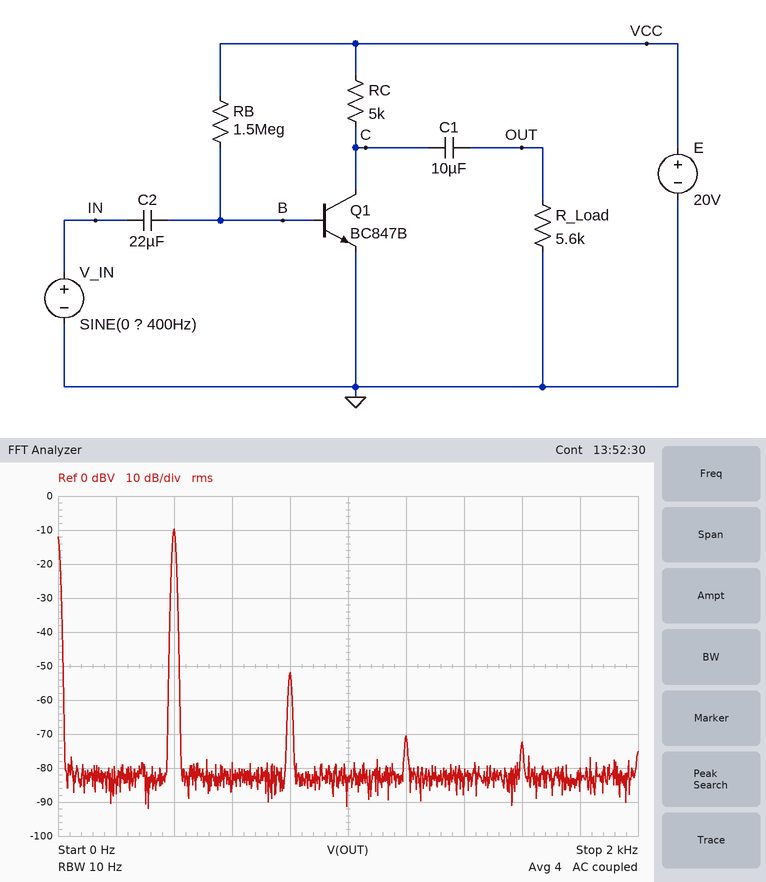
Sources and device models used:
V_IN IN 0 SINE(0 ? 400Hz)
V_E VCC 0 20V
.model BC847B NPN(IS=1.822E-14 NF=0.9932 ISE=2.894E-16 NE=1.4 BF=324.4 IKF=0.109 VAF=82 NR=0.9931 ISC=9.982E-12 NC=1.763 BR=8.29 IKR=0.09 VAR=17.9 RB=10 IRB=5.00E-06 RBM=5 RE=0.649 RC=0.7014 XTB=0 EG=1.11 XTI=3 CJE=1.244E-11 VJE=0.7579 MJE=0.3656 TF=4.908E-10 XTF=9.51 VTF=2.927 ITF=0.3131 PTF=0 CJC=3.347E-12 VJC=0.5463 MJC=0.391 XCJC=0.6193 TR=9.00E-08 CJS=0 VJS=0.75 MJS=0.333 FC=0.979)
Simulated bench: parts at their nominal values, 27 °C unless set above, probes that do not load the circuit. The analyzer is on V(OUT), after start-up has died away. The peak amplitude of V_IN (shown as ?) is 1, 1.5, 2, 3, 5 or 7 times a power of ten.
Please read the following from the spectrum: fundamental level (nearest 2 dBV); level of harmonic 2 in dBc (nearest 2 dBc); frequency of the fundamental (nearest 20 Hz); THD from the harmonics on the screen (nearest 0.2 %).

-10 dBV
-42 dBc
400 Hz
0.8 %
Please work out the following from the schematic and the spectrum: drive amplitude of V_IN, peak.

1.5 mV
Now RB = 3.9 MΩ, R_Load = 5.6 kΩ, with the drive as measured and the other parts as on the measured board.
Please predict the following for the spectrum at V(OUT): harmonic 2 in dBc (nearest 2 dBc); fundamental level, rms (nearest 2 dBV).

-38 dBc
-16 dBV
